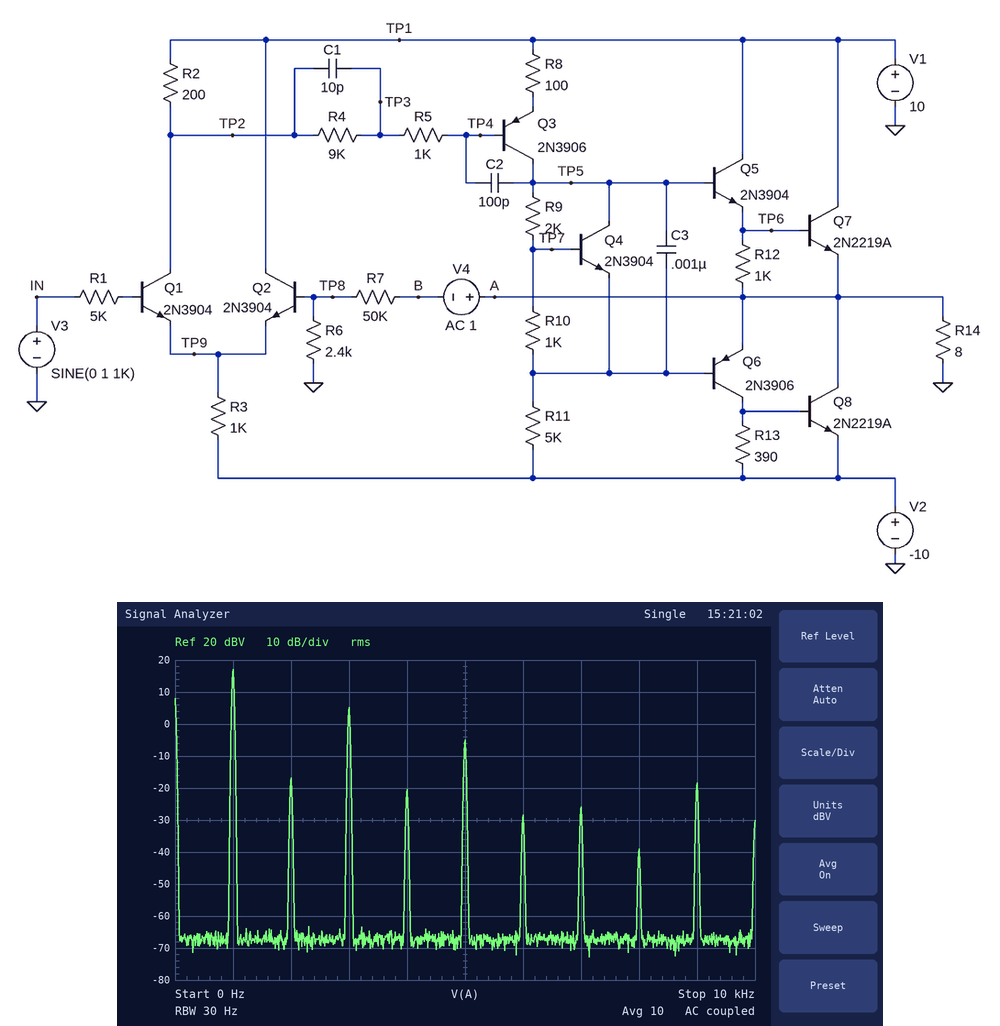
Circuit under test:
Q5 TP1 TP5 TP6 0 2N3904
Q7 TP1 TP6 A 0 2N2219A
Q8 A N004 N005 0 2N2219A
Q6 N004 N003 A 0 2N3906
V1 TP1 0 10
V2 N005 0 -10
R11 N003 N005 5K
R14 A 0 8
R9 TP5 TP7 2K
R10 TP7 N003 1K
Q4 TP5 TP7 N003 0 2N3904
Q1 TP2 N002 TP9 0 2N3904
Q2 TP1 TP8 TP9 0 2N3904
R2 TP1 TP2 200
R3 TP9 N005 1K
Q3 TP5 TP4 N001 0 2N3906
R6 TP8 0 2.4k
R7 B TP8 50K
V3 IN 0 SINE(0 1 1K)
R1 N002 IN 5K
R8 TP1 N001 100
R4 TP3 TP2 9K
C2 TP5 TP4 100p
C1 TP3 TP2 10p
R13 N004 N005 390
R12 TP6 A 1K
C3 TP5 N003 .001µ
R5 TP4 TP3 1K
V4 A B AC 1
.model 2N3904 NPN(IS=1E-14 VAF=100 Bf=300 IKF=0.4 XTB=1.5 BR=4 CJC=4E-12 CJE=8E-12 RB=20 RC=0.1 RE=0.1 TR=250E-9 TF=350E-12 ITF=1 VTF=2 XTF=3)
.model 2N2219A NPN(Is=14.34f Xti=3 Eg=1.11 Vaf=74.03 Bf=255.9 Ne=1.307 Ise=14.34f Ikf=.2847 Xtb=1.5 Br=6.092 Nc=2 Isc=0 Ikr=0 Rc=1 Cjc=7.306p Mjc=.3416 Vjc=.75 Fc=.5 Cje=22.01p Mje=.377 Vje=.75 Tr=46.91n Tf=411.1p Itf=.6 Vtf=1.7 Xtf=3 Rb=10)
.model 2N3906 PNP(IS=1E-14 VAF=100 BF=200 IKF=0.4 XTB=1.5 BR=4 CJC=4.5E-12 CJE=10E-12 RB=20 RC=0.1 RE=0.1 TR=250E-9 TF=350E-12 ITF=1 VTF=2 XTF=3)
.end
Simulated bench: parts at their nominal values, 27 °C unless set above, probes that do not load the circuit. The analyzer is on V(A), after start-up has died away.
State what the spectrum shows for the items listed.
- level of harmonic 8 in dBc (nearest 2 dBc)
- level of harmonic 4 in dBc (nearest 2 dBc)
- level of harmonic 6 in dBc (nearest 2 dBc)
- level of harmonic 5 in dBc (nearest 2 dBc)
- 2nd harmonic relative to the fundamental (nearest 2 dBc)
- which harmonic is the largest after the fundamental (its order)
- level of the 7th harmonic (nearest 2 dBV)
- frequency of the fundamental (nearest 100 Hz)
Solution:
-56 dBc
-38 dBc
-46 dBc
-22 dBc
-34 dBc
3
-26 dBV
1.0 kHz
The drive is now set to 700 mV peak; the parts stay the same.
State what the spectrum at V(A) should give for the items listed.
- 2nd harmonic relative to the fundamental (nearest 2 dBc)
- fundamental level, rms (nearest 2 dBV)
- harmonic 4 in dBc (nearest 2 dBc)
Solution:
-32 dBc
16 dBV
-42 dBc
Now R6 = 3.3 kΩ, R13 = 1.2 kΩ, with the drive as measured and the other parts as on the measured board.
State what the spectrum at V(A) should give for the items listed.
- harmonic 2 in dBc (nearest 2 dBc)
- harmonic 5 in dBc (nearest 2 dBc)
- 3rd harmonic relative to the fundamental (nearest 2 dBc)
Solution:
-52 dBc
-34 dBc
-14 dBc
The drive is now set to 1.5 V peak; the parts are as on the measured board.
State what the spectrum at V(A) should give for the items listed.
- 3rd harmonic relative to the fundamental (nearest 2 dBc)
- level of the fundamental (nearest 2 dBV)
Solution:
-10 dBc
18 dBV
